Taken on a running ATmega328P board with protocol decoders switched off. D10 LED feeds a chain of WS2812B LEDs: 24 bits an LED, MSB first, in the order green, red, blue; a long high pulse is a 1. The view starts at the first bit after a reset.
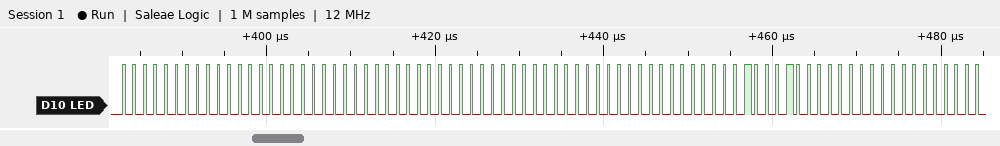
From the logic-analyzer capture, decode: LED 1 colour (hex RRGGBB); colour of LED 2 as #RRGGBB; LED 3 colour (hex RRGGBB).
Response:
#000000
#000000
#110000
